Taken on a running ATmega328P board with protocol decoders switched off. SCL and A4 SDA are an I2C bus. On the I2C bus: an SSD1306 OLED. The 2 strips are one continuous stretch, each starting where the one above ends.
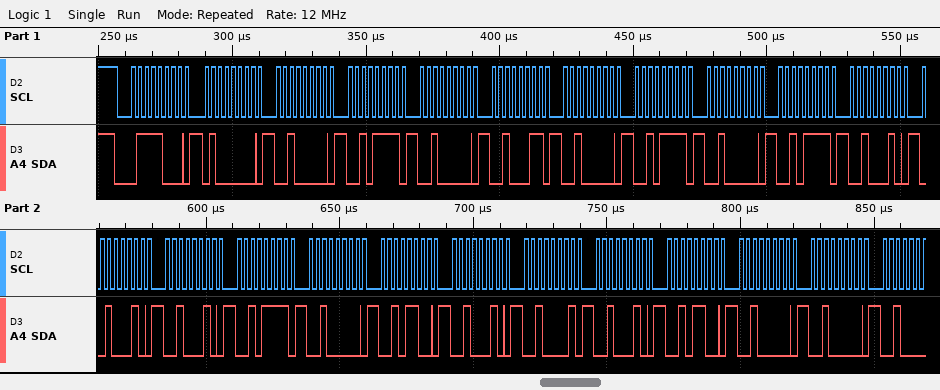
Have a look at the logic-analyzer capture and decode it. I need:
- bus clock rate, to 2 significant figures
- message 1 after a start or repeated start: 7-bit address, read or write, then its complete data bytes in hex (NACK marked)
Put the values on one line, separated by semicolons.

400 kHz; 0x3C write: 40 20 2F 20 23 20 2F 20 2F 22 22 22 2F 20 2C 22 21 22 2C 20 20
